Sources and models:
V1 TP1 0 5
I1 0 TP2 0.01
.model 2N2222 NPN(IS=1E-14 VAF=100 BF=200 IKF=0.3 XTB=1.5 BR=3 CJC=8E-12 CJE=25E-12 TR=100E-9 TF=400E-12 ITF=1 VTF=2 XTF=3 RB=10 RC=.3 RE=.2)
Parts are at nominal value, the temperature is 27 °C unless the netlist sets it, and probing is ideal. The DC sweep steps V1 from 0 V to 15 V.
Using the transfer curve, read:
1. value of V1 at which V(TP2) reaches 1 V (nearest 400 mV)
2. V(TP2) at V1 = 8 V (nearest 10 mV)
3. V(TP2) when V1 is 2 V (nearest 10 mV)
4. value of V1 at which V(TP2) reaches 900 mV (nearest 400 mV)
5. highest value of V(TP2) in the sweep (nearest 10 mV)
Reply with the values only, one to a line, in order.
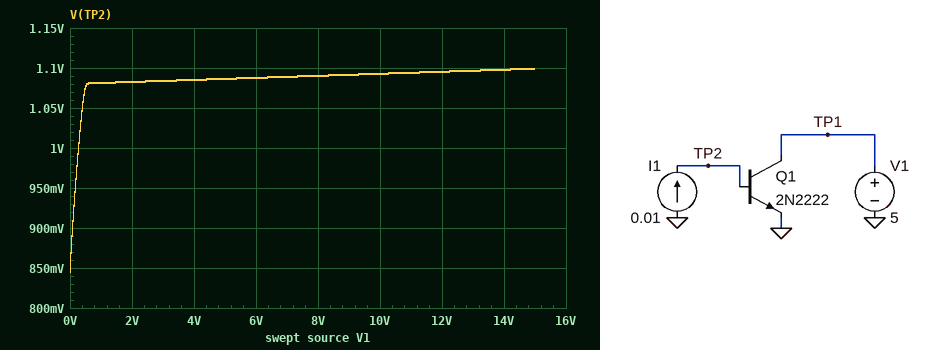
400 mV
1.09 V
1.08 V
0 V
1.10 V
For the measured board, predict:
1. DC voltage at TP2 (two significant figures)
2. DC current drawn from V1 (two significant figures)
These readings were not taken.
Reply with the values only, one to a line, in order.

1.1 V
660 mA
